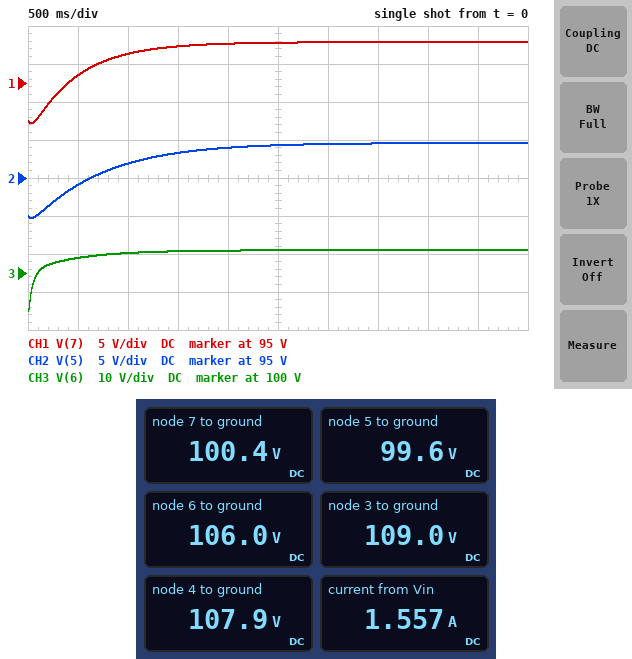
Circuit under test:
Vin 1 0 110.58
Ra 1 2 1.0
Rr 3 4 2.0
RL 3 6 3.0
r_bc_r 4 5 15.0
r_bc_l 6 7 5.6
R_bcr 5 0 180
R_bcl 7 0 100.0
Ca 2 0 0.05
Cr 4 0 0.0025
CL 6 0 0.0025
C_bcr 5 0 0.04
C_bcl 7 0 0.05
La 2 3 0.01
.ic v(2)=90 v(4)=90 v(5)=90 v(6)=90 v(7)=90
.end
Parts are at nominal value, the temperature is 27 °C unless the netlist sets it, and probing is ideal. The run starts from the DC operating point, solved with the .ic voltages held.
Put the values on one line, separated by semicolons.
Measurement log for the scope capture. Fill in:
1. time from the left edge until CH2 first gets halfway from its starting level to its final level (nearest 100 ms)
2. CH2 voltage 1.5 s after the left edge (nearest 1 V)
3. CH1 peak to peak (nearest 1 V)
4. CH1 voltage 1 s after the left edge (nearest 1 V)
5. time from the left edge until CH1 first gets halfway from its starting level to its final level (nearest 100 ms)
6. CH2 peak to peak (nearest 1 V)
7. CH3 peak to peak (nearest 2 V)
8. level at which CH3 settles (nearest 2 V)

600 ms; 98 V; 11 V; 99 V; 400 ms; 10 V; 16 V; 106 V
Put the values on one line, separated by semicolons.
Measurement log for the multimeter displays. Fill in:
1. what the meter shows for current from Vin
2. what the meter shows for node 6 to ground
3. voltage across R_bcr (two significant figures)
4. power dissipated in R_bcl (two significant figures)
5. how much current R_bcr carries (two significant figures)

1.557 A; 106.0 V; 100 V; 100 W; 550 mA
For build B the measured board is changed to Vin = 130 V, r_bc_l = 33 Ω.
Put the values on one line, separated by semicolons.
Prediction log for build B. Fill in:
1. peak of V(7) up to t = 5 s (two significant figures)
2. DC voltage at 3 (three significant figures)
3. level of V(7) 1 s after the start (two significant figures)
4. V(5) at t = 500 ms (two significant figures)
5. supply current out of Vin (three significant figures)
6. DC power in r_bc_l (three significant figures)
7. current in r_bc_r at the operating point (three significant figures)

94 V; 128 V; 91 V; 100 V; 1.60 A; 29.4 W; 652 mA
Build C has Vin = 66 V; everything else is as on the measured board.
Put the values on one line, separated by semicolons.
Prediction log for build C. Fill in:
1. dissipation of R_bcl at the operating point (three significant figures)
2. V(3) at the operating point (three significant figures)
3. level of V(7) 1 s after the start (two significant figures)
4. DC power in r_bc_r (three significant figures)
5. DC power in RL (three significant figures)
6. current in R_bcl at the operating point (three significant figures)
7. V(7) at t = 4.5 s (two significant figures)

35.9 W; 65.1 V; 64 V; 1.64 W; 1.08 W; 599 mA; 60 V
